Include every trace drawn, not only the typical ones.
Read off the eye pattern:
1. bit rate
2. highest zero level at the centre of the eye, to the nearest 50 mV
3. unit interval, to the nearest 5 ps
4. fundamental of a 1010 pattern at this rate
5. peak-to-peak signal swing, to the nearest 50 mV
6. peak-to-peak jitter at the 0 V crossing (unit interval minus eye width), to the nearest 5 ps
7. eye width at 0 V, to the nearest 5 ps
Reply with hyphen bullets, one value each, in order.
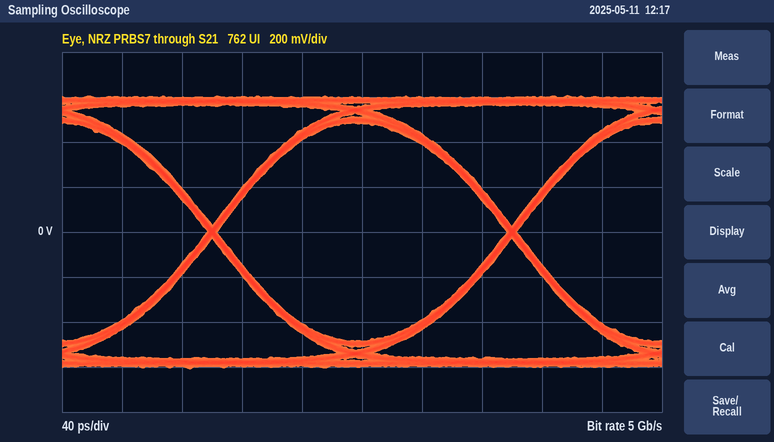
- 5 Gb/s
- -500 mV
- 200 ps
- 2.5 GHz
- 1.20 V
- 5 ps
- 195 ps
